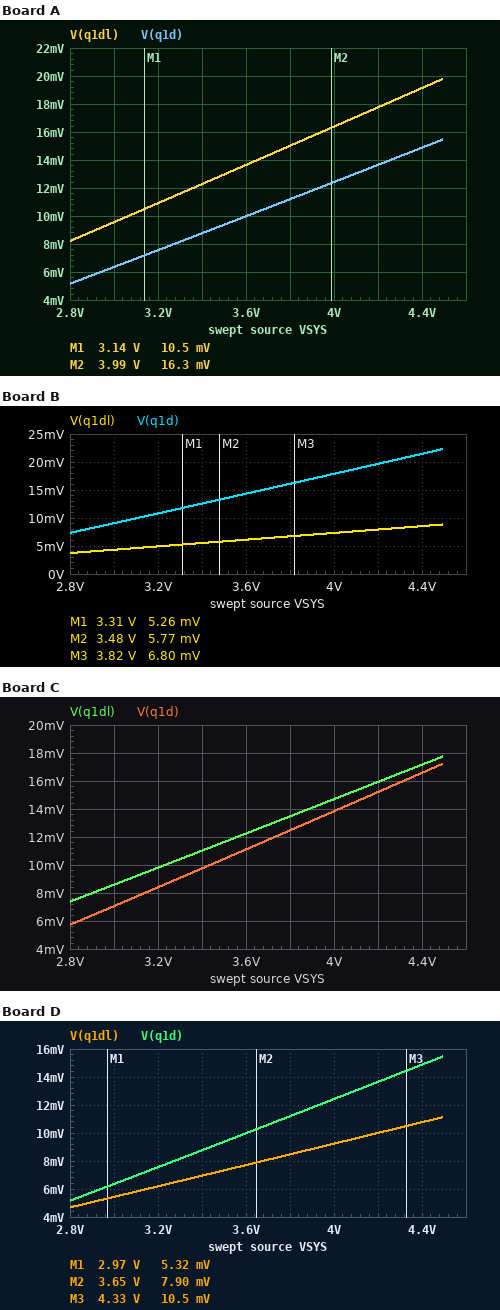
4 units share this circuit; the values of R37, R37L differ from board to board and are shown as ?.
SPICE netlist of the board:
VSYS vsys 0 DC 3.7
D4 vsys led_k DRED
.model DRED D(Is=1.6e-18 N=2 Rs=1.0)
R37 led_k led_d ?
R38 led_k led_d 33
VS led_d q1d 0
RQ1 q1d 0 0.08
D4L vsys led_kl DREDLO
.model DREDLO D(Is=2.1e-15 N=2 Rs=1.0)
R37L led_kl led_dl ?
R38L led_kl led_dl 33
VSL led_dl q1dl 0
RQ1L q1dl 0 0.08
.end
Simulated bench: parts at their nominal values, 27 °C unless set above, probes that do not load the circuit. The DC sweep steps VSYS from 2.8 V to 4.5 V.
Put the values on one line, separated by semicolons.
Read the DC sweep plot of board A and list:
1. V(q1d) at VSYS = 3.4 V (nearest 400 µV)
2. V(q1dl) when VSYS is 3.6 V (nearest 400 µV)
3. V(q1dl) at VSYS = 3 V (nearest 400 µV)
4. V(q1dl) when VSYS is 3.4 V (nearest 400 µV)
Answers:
8.8 mV; 13.6 mV; 9.6 mV; 12.4 mV
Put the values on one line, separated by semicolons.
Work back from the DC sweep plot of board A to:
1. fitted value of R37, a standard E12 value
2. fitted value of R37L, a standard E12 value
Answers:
18 Ω; 15 Ω
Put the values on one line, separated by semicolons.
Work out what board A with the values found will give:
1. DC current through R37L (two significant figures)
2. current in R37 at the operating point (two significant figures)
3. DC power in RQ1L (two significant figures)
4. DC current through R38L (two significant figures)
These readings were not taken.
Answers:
120 mA; 86 mA; 2.6 mW; 56 mA
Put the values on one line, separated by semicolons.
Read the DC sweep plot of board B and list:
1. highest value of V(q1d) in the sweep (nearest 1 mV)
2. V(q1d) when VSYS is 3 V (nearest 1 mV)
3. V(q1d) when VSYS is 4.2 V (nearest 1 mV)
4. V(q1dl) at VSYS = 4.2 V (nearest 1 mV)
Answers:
22 mV; 9 mV; 20 mV; 8 mV
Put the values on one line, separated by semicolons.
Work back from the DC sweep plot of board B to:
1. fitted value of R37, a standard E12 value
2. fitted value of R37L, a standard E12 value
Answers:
10 Ω; 100 Ω
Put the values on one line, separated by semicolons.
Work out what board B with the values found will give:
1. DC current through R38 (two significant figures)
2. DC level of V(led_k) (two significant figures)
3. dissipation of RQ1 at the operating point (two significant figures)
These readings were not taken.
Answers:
44 mA; 1.5 V; 2.9 mW
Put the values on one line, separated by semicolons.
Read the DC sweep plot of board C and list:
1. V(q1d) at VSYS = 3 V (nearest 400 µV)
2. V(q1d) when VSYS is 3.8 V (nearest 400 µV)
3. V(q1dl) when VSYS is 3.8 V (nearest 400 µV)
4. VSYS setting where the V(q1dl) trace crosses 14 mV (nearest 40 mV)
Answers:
7.2 mV; 12.4 mV; 13.6 mV; 3.88 V
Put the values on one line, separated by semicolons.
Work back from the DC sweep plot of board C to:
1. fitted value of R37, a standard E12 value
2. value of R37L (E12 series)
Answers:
15 Ω; 18 Ω
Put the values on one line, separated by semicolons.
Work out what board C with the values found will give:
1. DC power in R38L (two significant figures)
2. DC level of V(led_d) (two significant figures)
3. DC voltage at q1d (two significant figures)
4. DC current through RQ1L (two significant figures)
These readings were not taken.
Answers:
110 mW; 12 mV; 12 mV; 160 mA
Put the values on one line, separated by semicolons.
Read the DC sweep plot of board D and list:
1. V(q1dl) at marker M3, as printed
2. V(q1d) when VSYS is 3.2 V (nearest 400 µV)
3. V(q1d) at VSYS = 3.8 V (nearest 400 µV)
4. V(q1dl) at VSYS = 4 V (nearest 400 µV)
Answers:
10.5 mV; 7.6 mV; 11.2 mV; 9.2 mV
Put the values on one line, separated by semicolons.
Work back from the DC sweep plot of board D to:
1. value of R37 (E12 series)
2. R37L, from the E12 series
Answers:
18 Ω; 47 Ω
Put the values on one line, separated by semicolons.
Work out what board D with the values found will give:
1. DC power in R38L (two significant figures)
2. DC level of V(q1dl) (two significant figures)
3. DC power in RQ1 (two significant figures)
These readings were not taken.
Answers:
120 mW; 8.1 mV; 1.4 mW
